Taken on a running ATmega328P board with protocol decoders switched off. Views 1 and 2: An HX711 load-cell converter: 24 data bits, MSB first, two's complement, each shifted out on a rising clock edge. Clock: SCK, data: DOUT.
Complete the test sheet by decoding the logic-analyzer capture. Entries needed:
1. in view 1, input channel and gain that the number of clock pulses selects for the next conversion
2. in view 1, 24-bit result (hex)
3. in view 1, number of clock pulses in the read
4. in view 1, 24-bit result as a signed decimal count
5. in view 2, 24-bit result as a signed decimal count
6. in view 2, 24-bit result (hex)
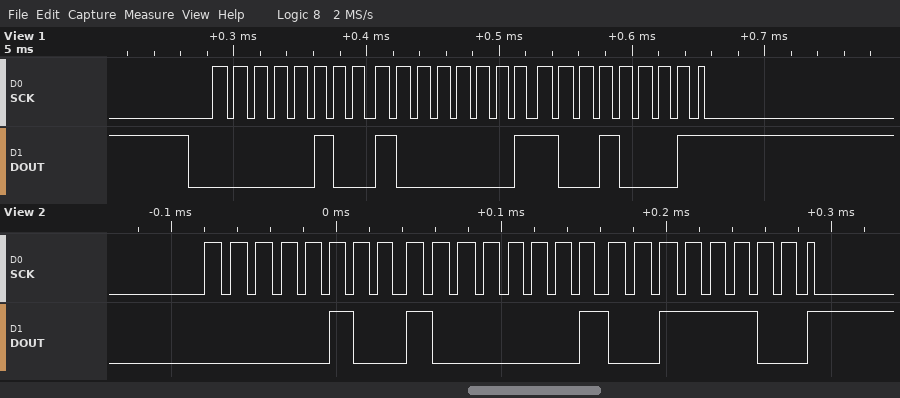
channel A, gain 128
0x048191
25
295313
295228
0x04813C
